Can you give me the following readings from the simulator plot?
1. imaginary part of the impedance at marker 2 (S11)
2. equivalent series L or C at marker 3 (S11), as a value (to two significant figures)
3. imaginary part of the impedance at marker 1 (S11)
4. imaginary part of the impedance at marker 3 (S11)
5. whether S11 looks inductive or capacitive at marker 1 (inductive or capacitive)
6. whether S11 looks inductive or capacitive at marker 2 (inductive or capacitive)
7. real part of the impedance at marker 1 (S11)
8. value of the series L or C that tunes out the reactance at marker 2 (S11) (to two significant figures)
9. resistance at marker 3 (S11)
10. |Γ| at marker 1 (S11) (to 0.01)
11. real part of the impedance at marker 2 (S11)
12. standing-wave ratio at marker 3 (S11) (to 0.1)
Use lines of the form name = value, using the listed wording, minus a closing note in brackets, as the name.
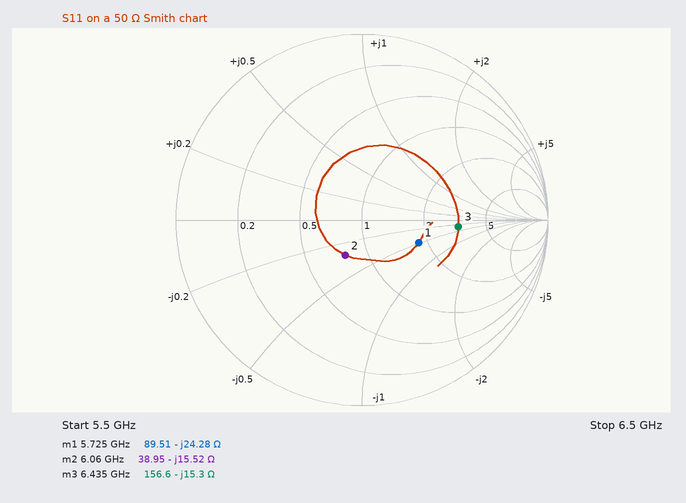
imaginary part of the impedance at marker 2 = -15.52 Ω
equivalent series L or C at marker 3 (S11), as a value = 1.6 pF
imaginary part of the impedance at marker 1 = -24.28 Ω
imaginary part of the impedance at marker 3 = -15.3 Ω
whether S11 looks inductive or capacitive at marker 1 = capacitive
whether S11 looks inductive or capacitive at marker 2 = capacitive
real part of the impedance at marker 1 = 89.51 Ω
value of the series L or C that tunes out the reactance at marker 2 (S11) = 410 pH
resistance at marker 3 = 156.6 Ω
|Γ| at marker 1 (S11) = 0.33
real part of the impedance at marker 2 = 38.95 Ω
standing-wave ratio at marker 3 (S11) = 3.2
